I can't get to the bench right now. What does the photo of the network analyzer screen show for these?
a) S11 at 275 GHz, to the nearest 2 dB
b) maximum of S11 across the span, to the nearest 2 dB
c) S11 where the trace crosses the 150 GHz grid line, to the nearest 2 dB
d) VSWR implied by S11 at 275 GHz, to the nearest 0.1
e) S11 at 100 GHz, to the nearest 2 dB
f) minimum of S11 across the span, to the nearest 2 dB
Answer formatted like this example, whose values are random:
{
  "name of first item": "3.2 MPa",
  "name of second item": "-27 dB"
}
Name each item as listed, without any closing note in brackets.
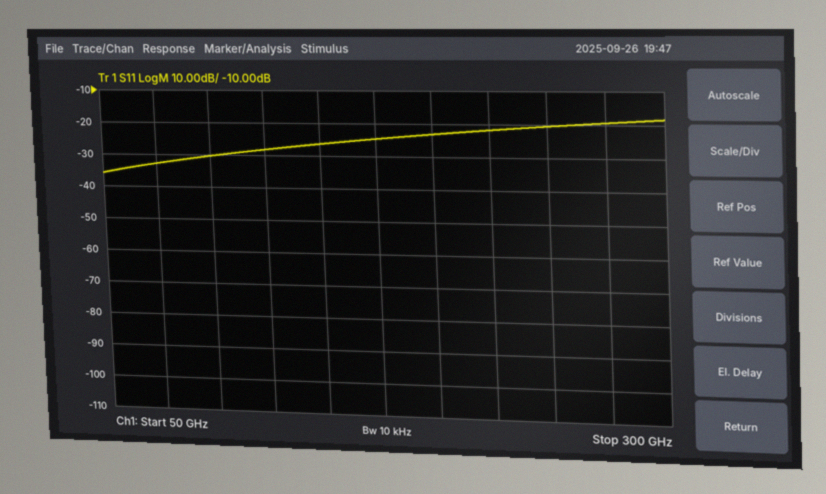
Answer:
{
  "S11 at 275 GHz, to the nearest 2 dB": "-20 dB",
  "maximum of S11 across the span, to the nearest 2 dB": "-18 dB",
  "S11 where the trace crosses the 150 GHz grid line, to the nearest 2 dB": "-26 dB",
  "VSWR implied by S11 at 275 GHz, to the nearest 0.1": "1.2",
  "S11 at 100 GHz, to the nearest 2 dB": "-30 dB",
  "minimum of S11 across the span, to the nearest 2 dB": "-36 dB"
}
